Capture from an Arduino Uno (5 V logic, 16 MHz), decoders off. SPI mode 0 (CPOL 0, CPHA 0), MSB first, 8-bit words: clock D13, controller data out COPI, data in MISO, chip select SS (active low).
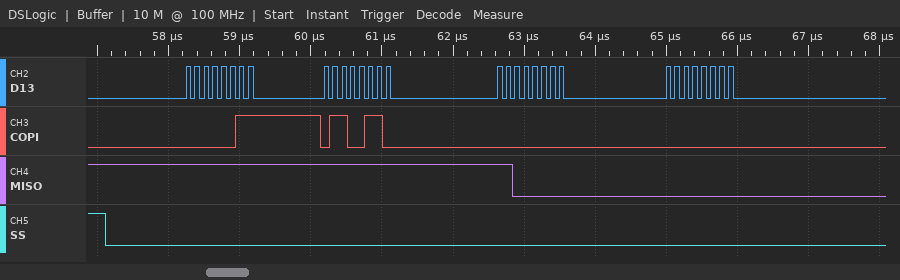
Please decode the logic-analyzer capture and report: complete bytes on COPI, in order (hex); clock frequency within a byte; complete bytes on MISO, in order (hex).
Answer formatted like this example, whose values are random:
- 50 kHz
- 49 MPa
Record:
- 0x03 0x66 0x00 0x00
- 8 MHz
- 0xFF 0xFF 0xC0 0x00
